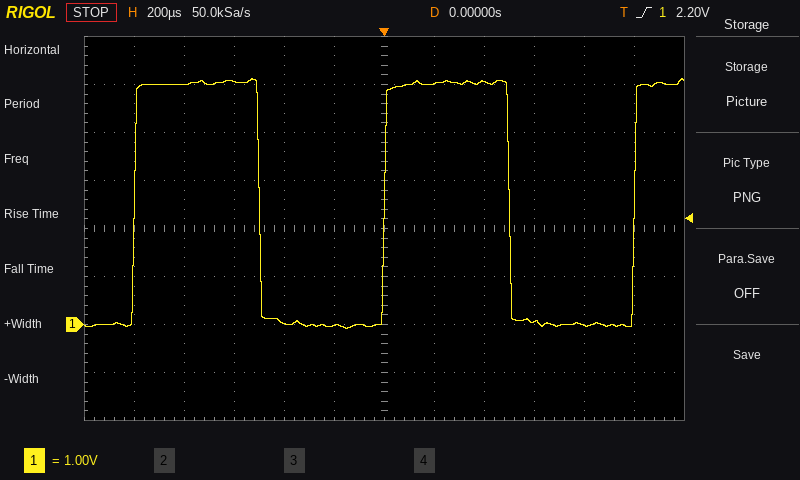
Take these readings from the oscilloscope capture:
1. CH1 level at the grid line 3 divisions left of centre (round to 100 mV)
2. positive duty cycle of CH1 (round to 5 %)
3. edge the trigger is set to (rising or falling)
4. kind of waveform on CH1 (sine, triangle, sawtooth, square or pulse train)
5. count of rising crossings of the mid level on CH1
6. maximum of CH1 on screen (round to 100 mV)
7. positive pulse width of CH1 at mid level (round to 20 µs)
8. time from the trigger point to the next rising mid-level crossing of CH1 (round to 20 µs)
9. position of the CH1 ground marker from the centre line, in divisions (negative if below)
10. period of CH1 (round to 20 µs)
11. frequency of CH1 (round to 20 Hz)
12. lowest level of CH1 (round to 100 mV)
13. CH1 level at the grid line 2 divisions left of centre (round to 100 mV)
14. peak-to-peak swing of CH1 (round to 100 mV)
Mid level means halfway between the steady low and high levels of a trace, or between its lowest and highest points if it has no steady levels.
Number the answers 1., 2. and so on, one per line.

1. 5.1 V
2. 50 %
3. rising
4. square
5. 3
6. 5.1 V
7. 500 µs
8. 1.00 ms
9. -2.0 div
10. 1.00 ms
11. 1.00 kHz
12. -100 mV
13. 0.0 V
14. 5.2 V
